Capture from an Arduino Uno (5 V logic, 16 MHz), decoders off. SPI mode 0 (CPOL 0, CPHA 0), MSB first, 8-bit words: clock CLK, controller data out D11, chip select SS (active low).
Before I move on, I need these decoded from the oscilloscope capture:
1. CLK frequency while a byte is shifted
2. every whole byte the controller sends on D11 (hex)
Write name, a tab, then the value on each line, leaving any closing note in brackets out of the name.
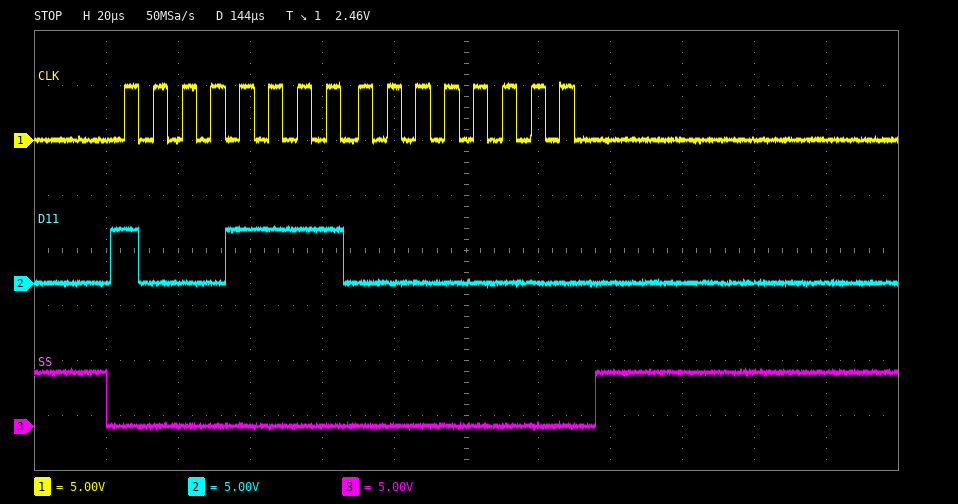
CLK frequency while a byte is shifted	125 kHz
every whole byte the controller sends on D11	8F 00
